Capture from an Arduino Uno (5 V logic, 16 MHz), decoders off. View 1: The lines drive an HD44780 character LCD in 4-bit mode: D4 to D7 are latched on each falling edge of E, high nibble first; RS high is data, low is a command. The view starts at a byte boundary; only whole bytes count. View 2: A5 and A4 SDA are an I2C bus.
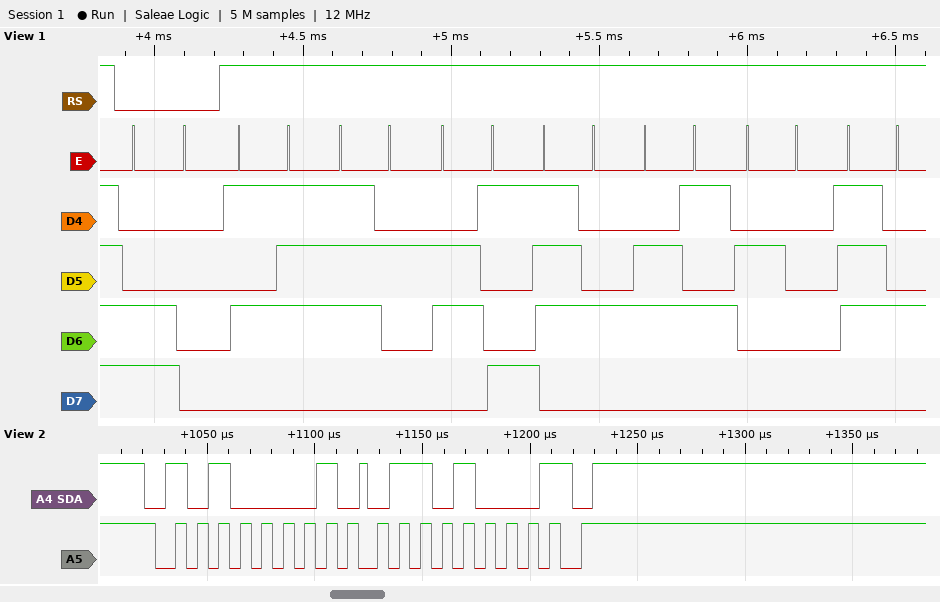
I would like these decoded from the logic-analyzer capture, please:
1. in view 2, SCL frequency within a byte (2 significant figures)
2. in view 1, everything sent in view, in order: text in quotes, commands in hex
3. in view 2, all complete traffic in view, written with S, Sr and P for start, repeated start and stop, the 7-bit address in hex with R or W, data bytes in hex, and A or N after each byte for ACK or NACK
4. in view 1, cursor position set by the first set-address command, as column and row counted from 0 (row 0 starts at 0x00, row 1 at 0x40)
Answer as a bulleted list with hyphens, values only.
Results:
- 100 kHz
- 0xC0 "Write t"
- S 50R A 68 N P
- column 0, row 1
